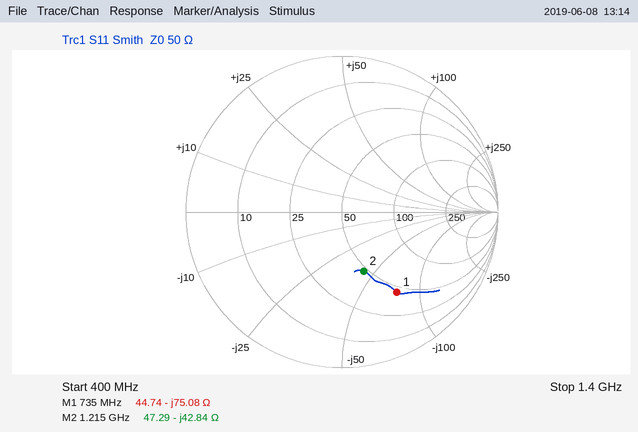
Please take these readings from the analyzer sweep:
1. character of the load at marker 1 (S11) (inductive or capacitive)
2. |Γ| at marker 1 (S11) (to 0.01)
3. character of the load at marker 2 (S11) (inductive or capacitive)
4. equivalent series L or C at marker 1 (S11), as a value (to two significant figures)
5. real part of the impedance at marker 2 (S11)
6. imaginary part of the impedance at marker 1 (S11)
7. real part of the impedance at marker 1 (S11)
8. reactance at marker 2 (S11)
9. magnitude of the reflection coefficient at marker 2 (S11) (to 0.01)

capacitive
0.62
capacitive
2.9 pF
47.29 Ω
-75.08 Ω
44.74 Ω
-42.84 Ω
0.40
